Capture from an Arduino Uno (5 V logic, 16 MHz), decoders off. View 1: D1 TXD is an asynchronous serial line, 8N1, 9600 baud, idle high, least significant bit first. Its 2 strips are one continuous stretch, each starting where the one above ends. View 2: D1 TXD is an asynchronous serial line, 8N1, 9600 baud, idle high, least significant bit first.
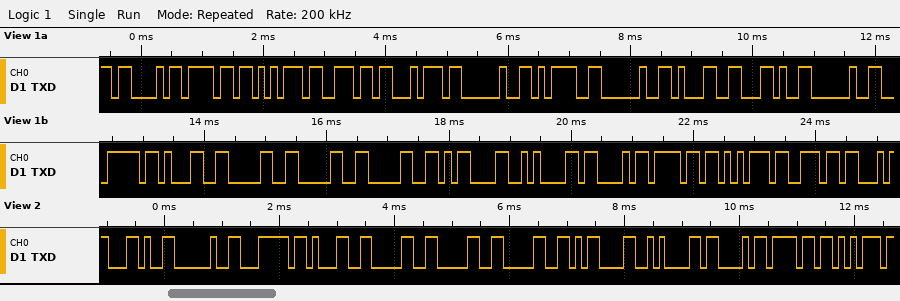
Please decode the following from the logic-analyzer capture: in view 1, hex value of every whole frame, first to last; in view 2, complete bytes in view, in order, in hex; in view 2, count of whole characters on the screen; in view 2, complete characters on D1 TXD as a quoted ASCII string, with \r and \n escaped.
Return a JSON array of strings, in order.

["43 6F 75 6E 74 20 3D 20 31 2C 20 7C 31 30 30 30 0D 0A 43 6F 75 6E", "2C 20 7C 31 30 30 30 0D 0A 43 6F 75", "12", "\", |1000\\r\\nCou\""]
